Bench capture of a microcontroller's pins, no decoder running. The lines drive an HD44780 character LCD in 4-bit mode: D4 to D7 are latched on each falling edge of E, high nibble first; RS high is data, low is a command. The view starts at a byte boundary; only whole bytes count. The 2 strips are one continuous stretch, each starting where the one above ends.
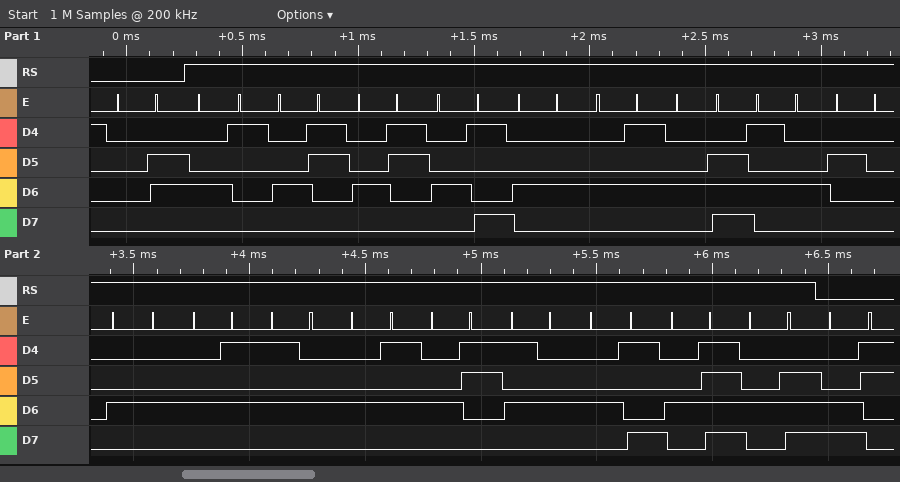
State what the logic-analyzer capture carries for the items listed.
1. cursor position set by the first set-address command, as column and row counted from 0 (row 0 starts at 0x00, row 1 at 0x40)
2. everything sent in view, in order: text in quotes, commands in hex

column 3, row 1
0x06 "ACCIDENT DETECTION" 0xC3
